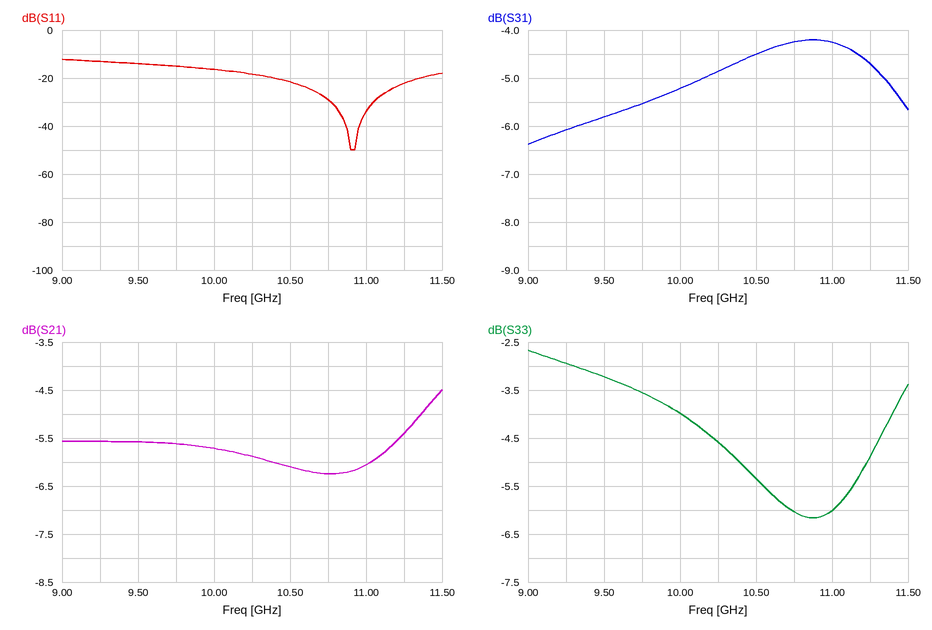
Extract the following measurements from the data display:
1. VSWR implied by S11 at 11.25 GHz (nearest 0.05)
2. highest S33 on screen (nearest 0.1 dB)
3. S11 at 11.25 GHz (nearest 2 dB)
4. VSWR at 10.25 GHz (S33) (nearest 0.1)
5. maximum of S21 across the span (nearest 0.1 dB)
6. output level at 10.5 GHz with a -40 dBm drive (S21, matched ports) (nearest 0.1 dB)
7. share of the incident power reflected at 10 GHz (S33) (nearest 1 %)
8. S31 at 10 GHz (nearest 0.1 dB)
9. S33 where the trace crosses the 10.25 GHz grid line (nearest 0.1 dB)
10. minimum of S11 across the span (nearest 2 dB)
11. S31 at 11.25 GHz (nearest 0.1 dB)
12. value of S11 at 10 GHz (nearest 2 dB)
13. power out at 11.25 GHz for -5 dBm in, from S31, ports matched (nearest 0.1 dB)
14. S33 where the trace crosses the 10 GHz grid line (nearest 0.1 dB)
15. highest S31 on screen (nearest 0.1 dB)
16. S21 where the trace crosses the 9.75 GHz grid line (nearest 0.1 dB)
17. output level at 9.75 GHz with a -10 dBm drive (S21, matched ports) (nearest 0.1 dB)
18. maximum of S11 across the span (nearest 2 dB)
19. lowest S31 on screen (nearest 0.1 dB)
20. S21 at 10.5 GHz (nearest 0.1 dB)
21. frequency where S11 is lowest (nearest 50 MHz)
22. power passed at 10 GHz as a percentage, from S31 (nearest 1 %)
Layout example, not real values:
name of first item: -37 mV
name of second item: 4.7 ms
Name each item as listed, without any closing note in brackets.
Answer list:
VSWR implied by S11 at 11.25 GHz: 1.15
highest S33 on screen: -2.7 dB
S11 at 11.25 GHz: -22 dB
VSWR at 10.25 GHz (S33): 3.9
maximum of S21 across the span: -4.5 dB
output level at 10.5 GHz with a -40 dBm drive (S21, matched ports): -46.1 dBm
share of the incident power reflected at 10 GHz (S33): 40 %
S31 at 10 GHz: -5.2 dB
S33 where the trace crosses the 10.25 GHz grid line: -4.6 dB
minimum of S11 across the span: -50 dB
S31 at 11.25 GHz: -4.7 dB
value of S11 at 10 GHz: -16 dB
power out at 11.25 GHz for -5 dBm in, from S31, ports matched: -9.7 dBm
S33 where the trace crosses the 10 GHz grid line: -4.0 dB
highest S31 on screen: -4.2 dB
S21 where the trace crosses the 9.75 GHz grid line: -5.6 dB
output level at 9.75 GHz with a -10 dBm drive (S21, matched ports): -15.6 dBm
maximum of S11 across the span: -12 dB
lowest S31 on screen: -6.4 dB
S21 at 10.5 GHz: -6.1 dB
frequency where S11 is lowest: 10.90 GHz
power passed at 10 GHz as a percentage, from S31: 30 %
